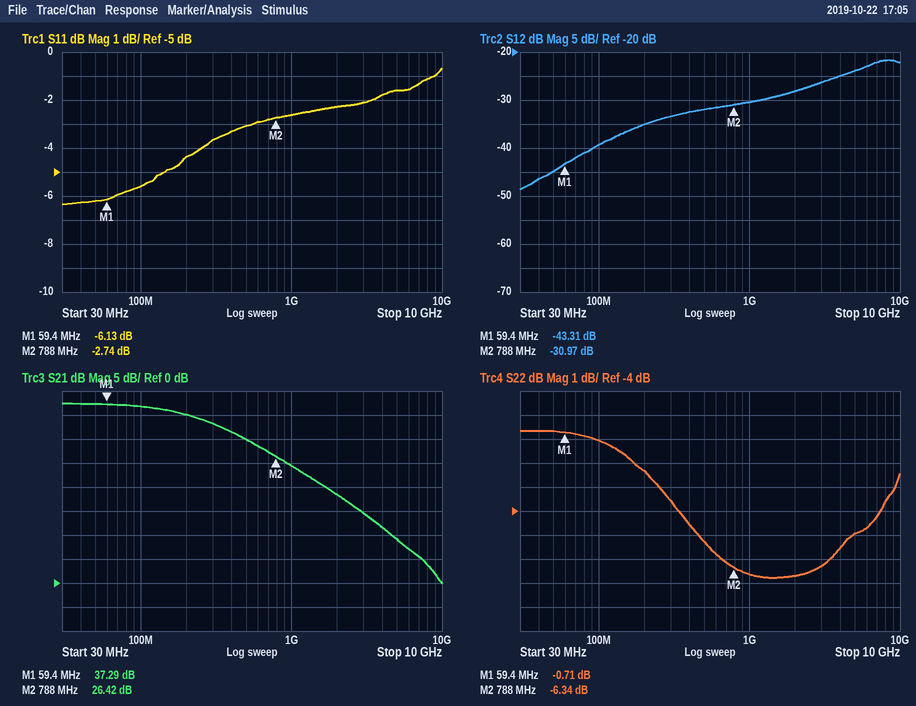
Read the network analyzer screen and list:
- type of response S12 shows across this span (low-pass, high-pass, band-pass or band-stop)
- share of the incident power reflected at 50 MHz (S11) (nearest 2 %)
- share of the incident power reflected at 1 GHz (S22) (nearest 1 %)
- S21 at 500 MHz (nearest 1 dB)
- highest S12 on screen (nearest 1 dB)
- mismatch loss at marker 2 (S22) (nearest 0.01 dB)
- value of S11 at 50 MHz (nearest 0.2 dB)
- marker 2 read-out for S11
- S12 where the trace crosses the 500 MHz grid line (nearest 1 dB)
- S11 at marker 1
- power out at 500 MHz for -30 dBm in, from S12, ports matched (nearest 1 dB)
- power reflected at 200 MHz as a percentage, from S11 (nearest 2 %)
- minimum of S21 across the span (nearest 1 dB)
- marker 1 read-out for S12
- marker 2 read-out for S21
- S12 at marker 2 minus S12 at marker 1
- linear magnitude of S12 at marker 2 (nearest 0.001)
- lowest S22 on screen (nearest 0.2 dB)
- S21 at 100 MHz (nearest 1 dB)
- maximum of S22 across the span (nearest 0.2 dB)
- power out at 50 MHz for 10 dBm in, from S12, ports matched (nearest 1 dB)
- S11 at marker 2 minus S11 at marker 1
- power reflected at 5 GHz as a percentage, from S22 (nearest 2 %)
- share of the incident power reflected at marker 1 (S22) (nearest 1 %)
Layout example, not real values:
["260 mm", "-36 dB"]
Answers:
["high-pass", "24 %", "22 %", "30 dB", "-22 dB", "1.15 dB", "-6.2 dB", "-2.74 dB", "-32 dB", "-6.13 dB", "-62 dBm", "36 %", "0 dB", "-43.31 dB", "26.42 dB", "12.34 dB", "0.028", "-6.8 dB", "37 dB", "-0.6 dB", "-35 dBm", "3.39 dB", "32 %", "85 %"]
